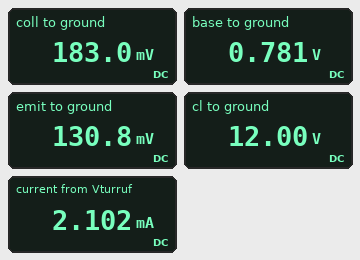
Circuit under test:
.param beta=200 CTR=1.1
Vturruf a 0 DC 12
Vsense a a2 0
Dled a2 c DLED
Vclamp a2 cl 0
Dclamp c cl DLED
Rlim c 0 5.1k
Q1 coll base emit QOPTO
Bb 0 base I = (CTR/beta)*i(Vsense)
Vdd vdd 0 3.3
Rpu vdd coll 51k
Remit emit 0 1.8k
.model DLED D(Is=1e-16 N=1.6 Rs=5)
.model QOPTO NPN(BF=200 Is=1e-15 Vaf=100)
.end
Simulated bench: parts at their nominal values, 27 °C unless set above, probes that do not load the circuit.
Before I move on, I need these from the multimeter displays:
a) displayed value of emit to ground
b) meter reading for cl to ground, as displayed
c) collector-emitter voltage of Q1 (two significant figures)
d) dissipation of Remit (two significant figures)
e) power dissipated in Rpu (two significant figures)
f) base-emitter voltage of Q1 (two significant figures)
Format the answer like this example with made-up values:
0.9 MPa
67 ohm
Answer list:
130.8 mV
12.00 V
52 mV
9.5 µW
190 µW
650 mV
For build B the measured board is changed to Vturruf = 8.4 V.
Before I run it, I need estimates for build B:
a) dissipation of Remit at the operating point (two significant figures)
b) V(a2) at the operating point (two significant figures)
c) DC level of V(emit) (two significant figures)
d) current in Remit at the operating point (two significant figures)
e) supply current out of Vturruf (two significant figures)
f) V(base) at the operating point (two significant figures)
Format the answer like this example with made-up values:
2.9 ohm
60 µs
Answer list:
8.5 µW
8.4 V
120 mV
69 µA
1.4 mA
770 mV
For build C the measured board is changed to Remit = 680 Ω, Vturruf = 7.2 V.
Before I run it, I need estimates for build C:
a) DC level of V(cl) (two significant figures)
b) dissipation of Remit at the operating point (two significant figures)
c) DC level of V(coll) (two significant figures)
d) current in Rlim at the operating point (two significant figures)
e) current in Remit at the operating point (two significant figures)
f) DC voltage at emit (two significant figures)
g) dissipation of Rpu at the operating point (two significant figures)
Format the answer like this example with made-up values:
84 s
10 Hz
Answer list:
7.2 V
3.2 µW
110 mV
1.2 mA
69 µA
47 mV
200 µW
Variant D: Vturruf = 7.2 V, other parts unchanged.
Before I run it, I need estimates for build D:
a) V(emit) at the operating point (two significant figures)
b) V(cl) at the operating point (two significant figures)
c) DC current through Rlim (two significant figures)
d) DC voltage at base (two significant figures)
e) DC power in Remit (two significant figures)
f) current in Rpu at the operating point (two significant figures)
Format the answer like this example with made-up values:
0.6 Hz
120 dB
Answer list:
120 mV
7.2 V
1.2 mA
770 mV
8.2 µW
61 µA
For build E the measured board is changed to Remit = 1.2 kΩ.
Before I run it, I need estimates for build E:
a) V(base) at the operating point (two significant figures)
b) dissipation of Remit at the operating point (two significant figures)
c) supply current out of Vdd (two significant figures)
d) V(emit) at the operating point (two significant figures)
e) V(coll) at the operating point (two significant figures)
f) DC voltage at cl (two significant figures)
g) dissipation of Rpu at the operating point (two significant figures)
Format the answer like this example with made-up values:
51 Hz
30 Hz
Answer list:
740 mV
6.5 µW
62 µA
88 mV
140 mV
12 V
200 µW
